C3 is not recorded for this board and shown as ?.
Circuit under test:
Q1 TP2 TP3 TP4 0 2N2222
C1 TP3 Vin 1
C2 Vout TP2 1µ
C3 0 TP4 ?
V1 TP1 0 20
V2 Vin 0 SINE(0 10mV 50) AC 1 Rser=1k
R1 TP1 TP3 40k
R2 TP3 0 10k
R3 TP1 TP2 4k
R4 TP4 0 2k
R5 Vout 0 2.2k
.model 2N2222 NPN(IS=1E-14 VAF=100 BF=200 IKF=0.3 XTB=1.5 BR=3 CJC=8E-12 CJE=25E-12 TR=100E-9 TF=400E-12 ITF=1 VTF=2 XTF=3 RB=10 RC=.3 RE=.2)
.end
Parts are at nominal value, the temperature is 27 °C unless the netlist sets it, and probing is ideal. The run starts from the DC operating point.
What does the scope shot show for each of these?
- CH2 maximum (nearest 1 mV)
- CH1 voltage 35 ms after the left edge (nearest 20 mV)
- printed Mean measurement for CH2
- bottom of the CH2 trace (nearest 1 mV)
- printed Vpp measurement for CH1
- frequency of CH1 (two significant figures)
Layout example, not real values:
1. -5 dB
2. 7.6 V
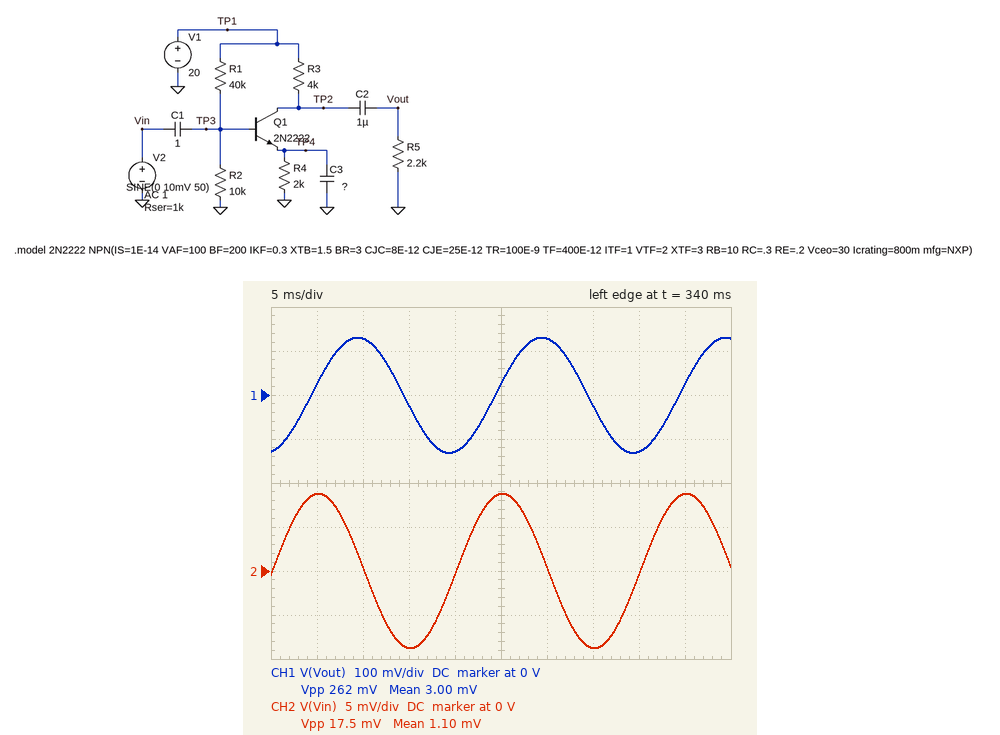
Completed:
1. 9 mV
2. -20 mV
3. 1.10 mV
4. -9 mV
5. 262 mV
6. 50 Hz
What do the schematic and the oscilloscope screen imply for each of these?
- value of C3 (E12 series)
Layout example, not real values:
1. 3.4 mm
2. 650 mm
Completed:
1. 39 µF
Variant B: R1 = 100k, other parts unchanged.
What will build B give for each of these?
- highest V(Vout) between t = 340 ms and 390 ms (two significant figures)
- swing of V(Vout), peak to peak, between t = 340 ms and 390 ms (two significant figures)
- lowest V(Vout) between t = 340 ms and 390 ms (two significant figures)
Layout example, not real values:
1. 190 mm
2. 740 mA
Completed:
1. 110 mV
2. 230 mV
3. -120 mV
